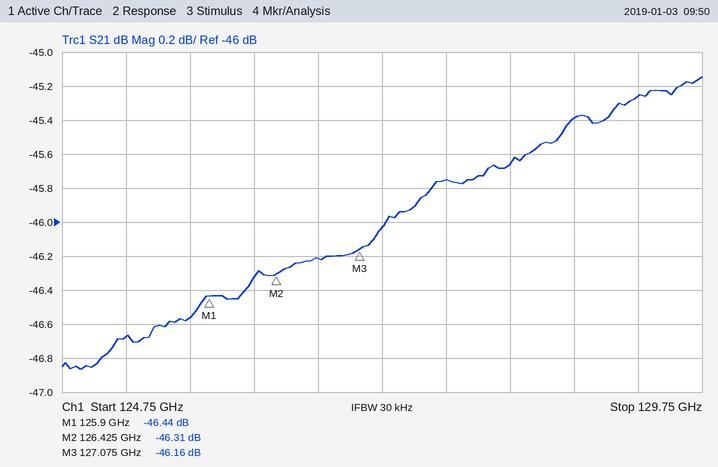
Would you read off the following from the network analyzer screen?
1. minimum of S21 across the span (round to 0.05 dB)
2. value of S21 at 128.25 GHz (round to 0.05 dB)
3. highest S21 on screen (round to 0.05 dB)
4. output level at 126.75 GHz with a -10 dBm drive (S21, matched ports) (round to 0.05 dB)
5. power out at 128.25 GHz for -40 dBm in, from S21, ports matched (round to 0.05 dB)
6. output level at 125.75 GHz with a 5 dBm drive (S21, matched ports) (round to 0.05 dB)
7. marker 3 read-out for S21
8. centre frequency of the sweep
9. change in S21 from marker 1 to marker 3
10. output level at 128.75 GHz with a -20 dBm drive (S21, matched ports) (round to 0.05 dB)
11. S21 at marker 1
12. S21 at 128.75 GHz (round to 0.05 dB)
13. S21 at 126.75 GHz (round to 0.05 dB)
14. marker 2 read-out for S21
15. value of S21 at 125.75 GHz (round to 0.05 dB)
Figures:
-46.85 dB
-45.65 dB
-45.15 dB
-56.20 dBm
-85.65 dBm
-41.55 dBm
-46.16 dB
127.25 GHz
0.28 dB
-65.40 dBm
-46.44 dB
-45.40 dB
-46.20 dB
-46.31 dB
-46.55 dB
